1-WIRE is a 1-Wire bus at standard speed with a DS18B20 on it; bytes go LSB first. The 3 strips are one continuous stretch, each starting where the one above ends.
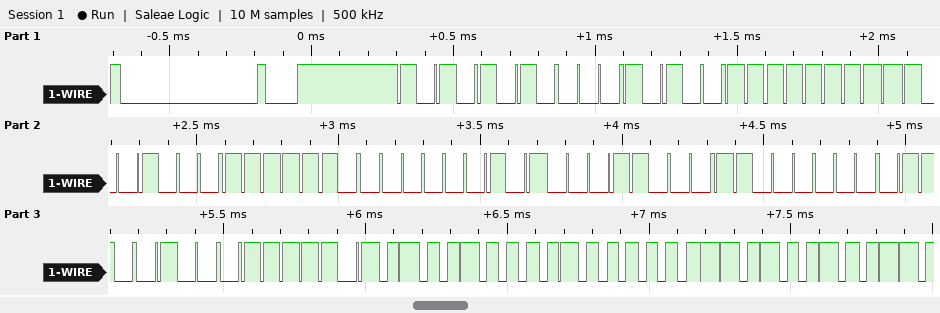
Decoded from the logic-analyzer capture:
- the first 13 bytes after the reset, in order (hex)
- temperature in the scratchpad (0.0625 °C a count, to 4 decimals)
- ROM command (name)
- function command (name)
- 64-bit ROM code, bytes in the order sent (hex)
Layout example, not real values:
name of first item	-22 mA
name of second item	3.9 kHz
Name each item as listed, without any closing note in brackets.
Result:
the first 13 bytes after the reset, in order	55 28 FF 13 3F A0 18 03 26 BE 12 02 4B
temperature in the scratchpad	33.1250 °C
ROM command	Match ROM
function command	Read Scratchpad
64-bit ROM code, bytes in the order sent	28 FF 13 3F A0 18 03 26
